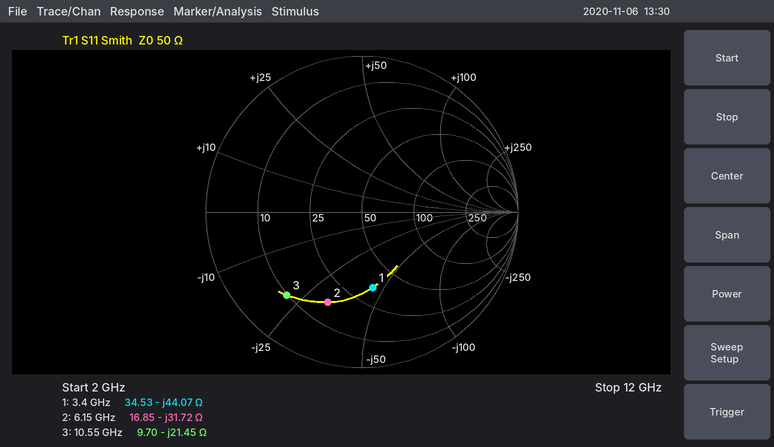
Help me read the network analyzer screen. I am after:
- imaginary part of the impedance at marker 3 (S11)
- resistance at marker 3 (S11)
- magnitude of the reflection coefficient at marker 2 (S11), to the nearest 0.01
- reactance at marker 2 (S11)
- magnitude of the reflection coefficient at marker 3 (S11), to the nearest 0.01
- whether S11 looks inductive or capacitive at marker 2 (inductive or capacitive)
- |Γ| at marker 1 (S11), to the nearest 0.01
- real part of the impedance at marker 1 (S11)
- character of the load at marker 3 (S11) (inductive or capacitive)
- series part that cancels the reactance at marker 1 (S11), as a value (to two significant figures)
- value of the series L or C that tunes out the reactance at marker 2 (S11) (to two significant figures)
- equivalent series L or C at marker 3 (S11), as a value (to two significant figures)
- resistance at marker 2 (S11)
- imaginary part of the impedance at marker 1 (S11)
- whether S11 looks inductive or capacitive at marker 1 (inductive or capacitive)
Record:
-21.45 Ω
9.70 Ω
0.62
-31.72 Ω
0.72
capacitive
0.49
34.53 Ω
capacitive
2.1 nH
820 pH
700 fF
16.85 Ω
-44.07 Ω
capacitive
